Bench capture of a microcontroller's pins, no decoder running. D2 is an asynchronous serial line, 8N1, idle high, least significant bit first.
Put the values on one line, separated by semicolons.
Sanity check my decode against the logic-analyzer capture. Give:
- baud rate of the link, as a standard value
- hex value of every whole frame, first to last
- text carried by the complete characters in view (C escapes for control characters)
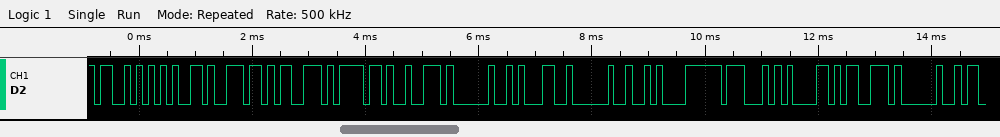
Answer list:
9600 baud; 53 65 6E 73 6F 72 20 31 20 0A 47 61 73 20; "Sensor 1 \nGas "
